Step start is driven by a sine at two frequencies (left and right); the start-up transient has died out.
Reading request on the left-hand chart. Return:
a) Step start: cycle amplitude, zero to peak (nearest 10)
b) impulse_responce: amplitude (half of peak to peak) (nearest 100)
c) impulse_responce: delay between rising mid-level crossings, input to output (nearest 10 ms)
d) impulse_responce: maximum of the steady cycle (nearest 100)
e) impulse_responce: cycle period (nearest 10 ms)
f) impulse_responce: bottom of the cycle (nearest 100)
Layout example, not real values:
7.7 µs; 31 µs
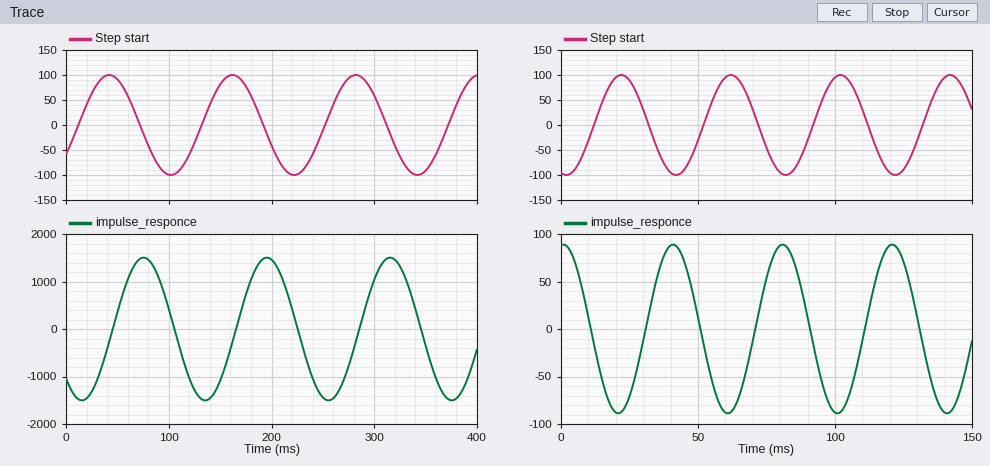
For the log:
100; 1500; 30 ms; 1500; 120 ms; -1500
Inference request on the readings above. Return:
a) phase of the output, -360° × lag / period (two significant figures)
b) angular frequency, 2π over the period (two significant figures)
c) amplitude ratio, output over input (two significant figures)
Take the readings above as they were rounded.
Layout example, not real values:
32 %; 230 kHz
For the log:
-90°; 0.052 rad/ms; 15
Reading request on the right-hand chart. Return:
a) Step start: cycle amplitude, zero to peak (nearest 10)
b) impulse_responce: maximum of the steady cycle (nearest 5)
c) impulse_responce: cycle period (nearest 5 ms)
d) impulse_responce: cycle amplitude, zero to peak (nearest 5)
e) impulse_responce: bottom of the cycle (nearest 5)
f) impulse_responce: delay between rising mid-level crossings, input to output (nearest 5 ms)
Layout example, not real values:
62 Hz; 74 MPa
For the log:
100; 90; 40 ms; 90; -90; 20 ms
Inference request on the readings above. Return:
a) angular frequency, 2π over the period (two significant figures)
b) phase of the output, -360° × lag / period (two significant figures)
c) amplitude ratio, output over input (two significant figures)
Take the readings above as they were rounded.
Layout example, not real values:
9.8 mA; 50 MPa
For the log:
0.16 rad/ms; -180°; 0.90
